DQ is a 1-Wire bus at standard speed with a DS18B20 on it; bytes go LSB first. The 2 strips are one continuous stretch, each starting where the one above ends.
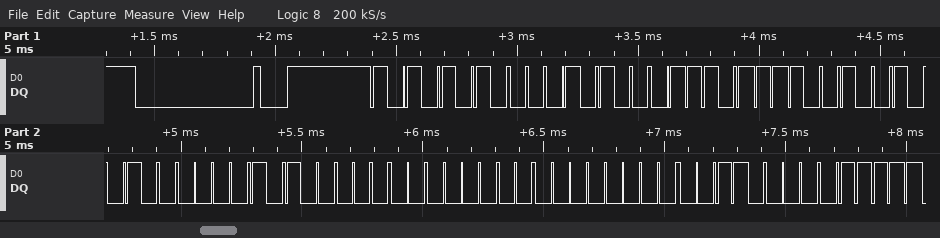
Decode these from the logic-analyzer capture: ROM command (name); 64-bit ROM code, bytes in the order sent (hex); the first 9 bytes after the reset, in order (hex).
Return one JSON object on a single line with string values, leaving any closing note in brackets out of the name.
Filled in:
{"ROM command": "Match ROM", "64-bit ROM code, bytes in the order sent": "28 EE 49 02 05 00 00 0C", "the first 9 bytes after the reset, in order": "55 28 EE 49 02 05 00 00 0C"}
